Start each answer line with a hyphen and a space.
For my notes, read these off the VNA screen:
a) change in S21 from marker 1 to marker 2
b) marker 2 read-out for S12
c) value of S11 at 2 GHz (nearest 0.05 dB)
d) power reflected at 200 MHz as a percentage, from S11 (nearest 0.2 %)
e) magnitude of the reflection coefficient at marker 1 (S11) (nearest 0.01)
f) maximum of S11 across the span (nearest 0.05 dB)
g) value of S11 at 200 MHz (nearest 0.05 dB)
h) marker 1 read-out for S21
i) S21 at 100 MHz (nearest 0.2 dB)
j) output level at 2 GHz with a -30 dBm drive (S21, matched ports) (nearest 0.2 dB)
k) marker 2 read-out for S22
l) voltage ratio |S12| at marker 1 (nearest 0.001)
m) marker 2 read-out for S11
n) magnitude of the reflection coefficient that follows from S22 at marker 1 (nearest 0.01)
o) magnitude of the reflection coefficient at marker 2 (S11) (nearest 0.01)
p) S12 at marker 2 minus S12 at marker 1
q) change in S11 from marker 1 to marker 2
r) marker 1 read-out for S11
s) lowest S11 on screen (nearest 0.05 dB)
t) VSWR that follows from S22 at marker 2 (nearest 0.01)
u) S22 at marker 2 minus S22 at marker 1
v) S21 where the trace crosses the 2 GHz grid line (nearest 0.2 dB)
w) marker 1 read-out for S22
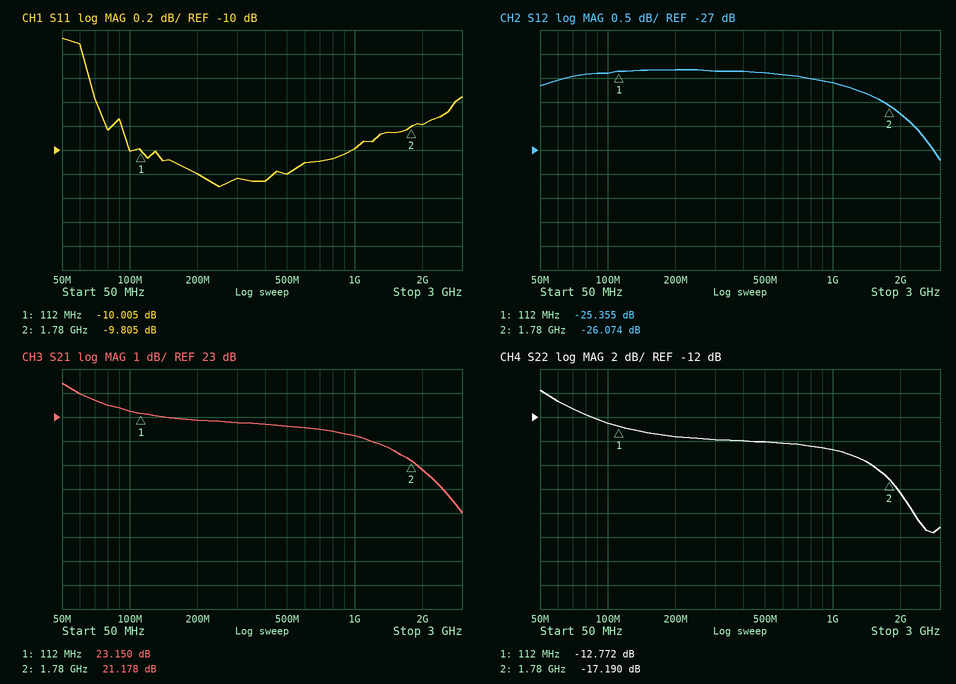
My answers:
- -1.972 dB
- -26.074 dB
- -9.80 dB
- 9.6 %
- 0.32
- -9.05 dB
- -10.20 dB
- 23.150 dB
- 23.2 dB
- -9.2 dBm
- -17.190 dB
- 0.054
- -9.805 dB
- 0.23
- 0.32
- -0.719 dB
- 0.200 dB
- -10.005 dB
- -10.30 dB
- 1.32
- -4.418 dB
- 20.8 dB
- -12.772 dB
